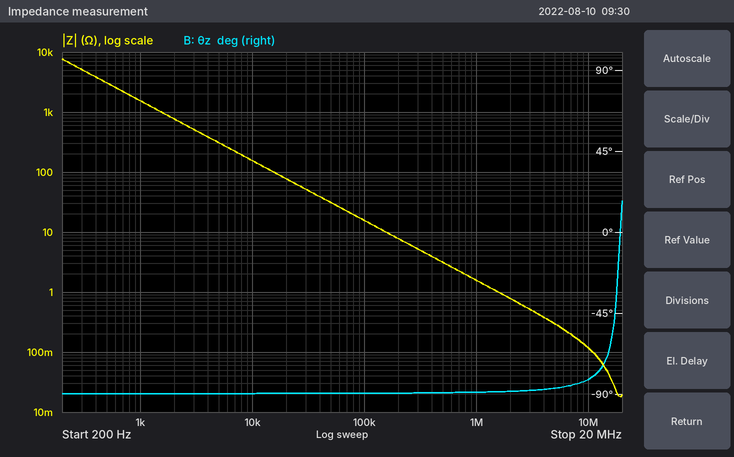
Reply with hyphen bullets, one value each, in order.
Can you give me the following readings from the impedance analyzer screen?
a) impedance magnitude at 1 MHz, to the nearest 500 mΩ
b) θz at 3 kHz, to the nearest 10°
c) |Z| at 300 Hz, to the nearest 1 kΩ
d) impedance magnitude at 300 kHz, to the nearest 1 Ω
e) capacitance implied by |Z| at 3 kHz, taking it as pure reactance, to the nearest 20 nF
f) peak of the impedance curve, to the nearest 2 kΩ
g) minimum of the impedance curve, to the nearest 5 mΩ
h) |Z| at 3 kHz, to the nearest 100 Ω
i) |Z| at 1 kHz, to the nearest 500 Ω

- 1.5 Ω
- -90°
- 5 kΩ
- 5 Ω
- 100 nF
- 8 kΩ
- 20 mΩ
- 500 Ω
- 1.5 kΩ
